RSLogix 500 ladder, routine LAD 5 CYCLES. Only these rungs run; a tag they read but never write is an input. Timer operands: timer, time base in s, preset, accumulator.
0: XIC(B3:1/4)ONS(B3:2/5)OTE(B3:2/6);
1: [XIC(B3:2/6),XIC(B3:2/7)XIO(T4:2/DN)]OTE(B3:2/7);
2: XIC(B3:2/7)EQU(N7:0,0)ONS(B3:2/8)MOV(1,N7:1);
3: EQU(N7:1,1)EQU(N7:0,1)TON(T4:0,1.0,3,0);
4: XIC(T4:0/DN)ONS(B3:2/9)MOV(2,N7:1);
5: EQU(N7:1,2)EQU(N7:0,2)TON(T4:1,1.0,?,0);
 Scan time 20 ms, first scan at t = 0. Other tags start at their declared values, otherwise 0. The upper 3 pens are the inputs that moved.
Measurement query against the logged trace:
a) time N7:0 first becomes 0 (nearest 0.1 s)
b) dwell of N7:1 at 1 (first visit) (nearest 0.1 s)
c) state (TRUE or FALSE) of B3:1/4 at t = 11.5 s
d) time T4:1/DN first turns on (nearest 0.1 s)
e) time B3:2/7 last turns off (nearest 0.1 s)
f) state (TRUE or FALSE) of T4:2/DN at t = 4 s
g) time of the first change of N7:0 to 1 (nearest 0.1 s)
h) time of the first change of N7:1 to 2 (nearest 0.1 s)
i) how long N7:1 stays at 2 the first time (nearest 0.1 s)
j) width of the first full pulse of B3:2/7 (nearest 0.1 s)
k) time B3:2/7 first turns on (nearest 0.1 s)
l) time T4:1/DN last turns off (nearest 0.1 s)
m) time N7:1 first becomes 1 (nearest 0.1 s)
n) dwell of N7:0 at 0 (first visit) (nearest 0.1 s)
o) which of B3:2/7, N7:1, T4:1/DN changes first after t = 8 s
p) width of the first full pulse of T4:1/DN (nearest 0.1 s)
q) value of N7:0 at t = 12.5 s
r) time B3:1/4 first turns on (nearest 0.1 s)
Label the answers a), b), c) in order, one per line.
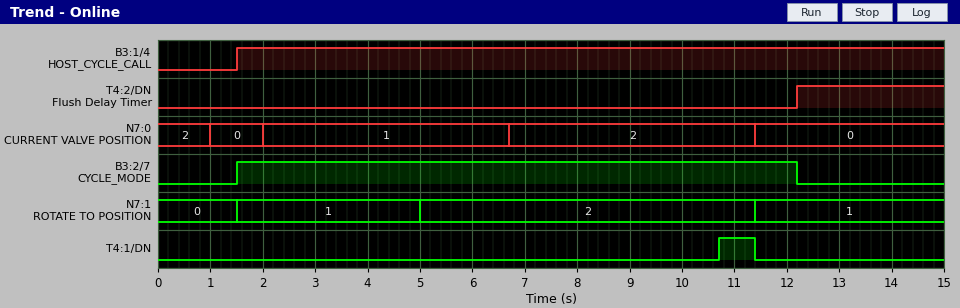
a) 1.0 s
b) 3.5 s
c) TRUE
d) 10.7 s
e) 12.2 s
f) FALSE
g) 2.0 s
h) 5.0 s
i) 6.4 s
j) 10.7 s
k) 1.5 s
l) 11.4 s
m) 1.5 s
n) 1.0 s
o) T4:1/DN
p) 0.7 s
q) 0
r) 1.5 s
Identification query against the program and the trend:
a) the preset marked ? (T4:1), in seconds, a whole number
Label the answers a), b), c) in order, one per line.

a) 4 s
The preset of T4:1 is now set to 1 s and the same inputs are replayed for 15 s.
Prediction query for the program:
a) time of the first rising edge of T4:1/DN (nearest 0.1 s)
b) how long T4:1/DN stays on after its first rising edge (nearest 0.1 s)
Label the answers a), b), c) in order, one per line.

a) 7.7 s
b) 3.7 s
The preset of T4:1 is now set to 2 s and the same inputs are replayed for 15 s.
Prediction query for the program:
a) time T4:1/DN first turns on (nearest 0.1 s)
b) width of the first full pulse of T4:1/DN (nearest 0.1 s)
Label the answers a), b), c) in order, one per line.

a) 8.7 s
b) 2.7 s
